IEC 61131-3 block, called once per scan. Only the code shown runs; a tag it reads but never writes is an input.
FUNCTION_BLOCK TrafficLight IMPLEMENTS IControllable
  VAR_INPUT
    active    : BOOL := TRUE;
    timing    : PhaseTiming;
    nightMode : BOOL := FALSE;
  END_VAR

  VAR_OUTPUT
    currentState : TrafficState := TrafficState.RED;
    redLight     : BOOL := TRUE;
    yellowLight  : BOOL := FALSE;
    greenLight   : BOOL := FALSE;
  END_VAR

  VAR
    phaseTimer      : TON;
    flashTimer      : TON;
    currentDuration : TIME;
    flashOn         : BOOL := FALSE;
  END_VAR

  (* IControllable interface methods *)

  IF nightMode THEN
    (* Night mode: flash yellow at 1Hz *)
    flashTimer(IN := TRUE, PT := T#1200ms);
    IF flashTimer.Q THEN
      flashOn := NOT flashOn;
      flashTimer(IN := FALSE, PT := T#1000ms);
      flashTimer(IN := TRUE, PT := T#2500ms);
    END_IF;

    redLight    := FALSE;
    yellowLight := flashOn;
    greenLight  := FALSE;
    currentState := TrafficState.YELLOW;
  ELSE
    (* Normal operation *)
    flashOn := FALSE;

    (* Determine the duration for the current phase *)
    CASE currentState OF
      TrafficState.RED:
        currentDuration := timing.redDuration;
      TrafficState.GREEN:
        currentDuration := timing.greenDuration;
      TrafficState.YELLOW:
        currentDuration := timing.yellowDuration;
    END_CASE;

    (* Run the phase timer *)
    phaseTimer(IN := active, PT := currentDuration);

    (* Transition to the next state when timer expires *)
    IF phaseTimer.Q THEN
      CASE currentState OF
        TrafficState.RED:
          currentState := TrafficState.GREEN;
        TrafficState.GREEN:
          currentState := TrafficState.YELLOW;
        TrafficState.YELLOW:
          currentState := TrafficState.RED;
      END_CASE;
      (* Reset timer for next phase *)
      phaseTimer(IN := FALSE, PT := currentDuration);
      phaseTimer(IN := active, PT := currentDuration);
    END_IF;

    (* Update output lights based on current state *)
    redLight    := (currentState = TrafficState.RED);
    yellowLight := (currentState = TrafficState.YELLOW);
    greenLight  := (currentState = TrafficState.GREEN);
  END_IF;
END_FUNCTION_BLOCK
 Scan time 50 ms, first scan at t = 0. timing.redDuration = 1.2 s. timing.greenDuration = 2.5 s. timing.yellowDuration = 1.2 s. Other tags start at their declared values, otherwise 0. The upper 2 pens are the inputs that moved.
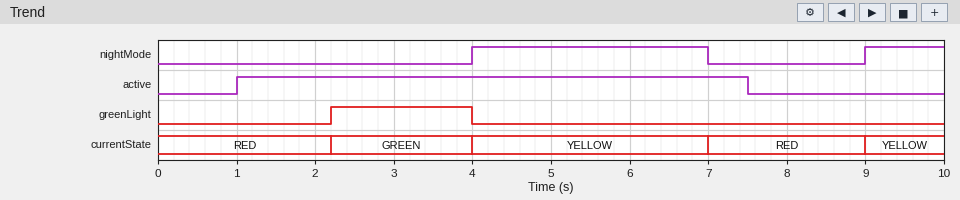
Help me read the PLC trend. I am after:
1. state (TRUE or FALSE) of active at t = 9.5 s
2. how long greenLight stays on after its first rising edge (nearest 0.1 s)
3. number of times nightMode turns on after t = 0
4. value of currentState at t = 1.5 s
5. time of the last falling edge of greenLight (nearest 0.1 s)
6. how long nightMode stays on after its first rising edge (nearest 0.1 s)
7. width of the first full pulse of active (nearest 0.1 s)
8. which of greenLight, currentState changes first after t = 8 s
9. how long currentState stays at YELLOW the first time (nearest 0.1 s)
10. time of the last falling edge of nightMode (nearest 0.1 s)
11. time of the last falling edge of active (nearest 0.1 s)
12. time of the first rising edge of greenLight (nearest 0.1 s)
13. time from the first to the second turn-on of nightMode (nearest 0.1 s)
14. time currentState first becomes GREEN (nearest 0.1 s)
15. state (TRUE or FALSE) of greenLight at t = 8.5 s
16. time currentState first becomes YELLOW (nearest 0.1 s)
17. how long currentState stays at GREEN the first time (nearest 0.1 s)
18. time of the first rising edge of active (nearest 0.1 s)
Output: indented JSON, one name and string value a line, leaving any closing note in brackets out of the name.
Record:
{
  "state (TRUE or FALSE) of active at t = 9.5 s": "FALSE",
  "how long greenLight stays on after its first rising edge": "1.8 s",
  "number of times nightMode turns on after t = 0": "2",
  "value of currentState at t = 1.5 s": "RED",
  "time of the last falling edge of greenLight": "4.0 s",
  "how long nightMode stays on after its first rising edge": "3.0 s",
  "width of the first full pulse of active": "6.5 s",
  "which of greenLight, currentState changes first after t = 8 s": "currentState",
  "how long currentState stays at YELLOW the first time": "3.0 s",
  "time of the last falling edge of nightMode": "7.0 s",
  "time of the last falling edge of active": "7.5 s",
  "time of the first rising edge of greenLight": "2.2 s",
  "time from the first to the second turn-on of nightMode": "5.0 s",
  "time currentState first becomes GREEN": "2.2 s",
  "state (TRUE or FALSE) of greenLight at t = 8.5 s": "FALSE",
  "time currentState first becomes YELLOW": "4.0 s",
  "how long currentState stays at GREEN the first time": "1.8 s",
  "time of the first rising edge of active": "1.0 s"
}
